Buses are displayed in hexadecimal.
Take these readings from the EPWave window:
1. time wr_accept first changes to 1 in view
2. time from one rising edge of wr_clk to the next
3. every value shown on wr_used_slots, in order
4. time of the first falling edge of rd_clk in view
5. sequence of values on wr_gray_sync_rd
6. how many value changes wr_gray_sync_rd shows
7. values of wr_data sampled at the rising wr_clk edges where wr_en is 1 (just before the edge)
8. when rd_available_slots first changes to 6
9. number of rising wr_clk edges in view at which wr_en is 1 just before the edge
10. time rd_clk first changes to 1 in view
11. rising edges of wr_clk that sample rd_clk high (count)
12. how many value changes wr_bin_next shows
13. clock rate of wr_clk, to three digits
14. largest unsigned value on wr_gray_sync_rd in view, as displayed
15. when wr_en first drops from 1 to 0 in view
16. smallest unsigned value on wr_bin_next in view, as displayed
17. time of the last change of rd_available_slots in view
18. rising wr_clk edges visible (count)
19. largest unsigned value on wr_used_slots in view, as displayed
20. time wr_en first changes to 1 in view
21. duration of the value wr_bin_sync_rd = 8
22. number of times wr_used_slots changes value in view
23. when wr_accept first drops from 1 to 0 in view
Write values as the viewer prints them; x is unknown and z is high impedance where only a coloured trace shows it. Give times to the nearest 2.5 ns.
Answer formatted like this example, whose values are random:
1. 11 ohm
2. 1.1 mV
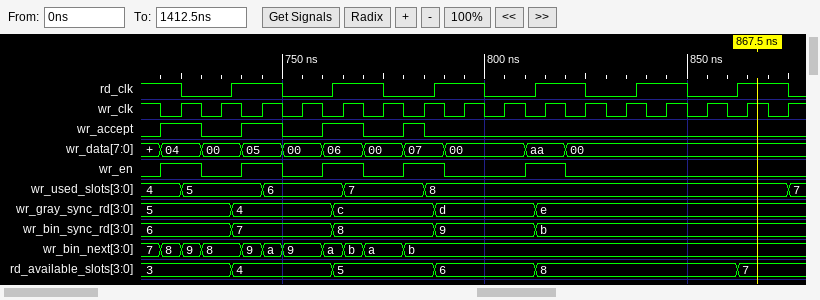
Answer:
1. 720 ns
2. 10 ns
3. 4, 5, 6, 7, 8, 7
4. 725 ns
5. 5, 4, c, d, e
6. 4
7. 04, 05, 06, 07, aa
8. 787.5 ns
9. 5
10. 737.5 ns
11. 10
12. 10
13. 100 MHz
14. e
15. 730 ns
16. 7
17. 862.5 ns
18. 16
19. 8
20. 720 ns
21. 25 ns
22. 5
23. 730 ns
